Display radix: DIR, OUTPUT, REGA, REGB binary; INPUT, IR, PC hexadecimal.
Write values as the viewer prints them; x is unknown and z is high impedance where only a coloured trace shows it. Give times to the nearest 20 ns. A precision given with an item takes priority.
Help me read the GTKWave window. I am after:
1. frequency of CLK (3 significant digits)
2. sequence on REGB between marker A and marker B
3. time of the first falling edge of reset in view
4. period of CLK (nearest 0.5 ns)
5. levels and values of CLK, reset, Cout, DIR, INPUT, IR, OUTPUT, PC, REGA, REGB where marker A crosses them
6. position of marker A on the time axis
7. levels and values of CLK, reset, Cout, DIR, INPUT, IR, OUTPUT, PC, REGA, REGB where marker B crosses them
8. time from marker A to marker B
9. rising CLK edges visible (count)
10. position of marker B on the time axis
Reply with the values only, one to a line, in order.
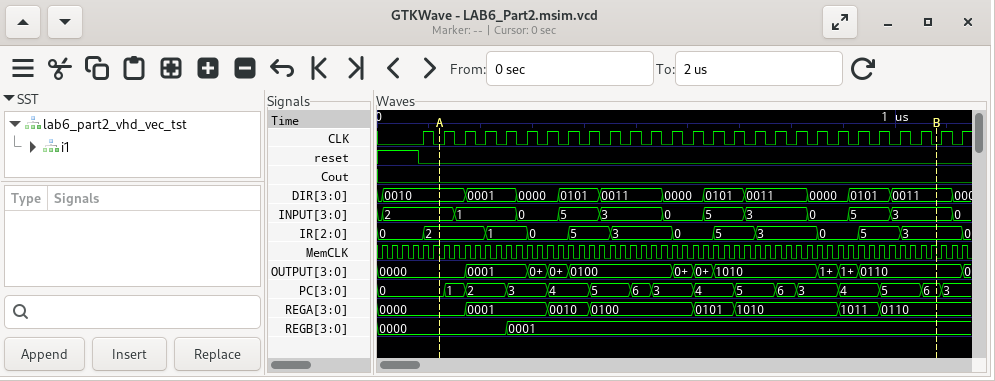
25.0 MHz
0000, 0001
80 ns
40 ns
CLK=0, reset=0, Cout=0, DIR=0010, INPUT=2, IR=2, OUTPUT=0000, PC=0, REGA=0000, REGB=0000
120 ns
CLK=0, reset=0, Cout=0, DIR=0011, INPUT=3, IR=3, OUTPUT=0110, PC=6, REGA=0110, REGB=0001
960 ns
27
1080 ns
